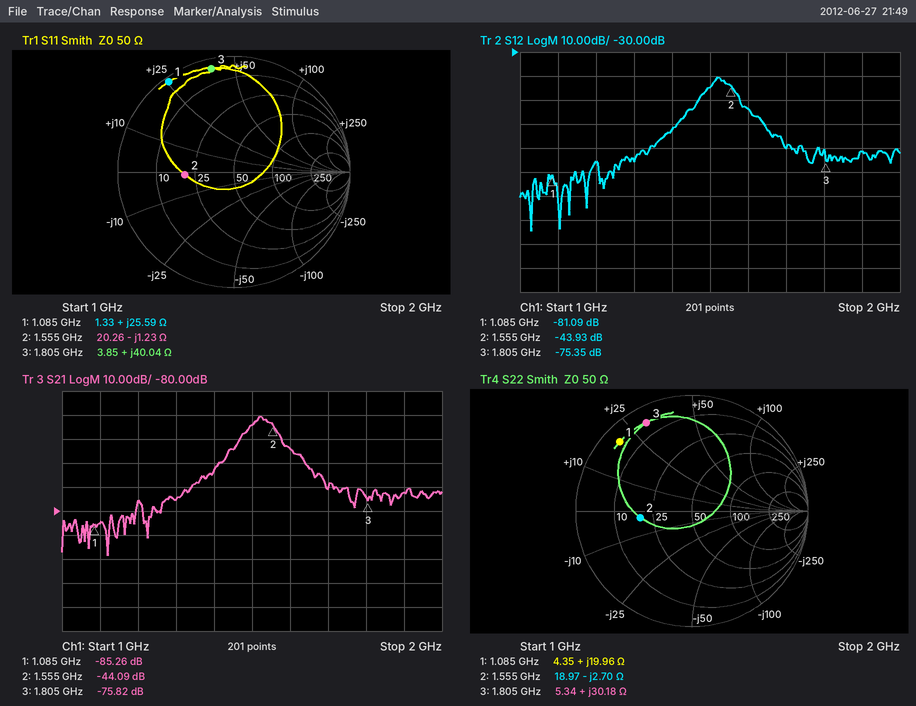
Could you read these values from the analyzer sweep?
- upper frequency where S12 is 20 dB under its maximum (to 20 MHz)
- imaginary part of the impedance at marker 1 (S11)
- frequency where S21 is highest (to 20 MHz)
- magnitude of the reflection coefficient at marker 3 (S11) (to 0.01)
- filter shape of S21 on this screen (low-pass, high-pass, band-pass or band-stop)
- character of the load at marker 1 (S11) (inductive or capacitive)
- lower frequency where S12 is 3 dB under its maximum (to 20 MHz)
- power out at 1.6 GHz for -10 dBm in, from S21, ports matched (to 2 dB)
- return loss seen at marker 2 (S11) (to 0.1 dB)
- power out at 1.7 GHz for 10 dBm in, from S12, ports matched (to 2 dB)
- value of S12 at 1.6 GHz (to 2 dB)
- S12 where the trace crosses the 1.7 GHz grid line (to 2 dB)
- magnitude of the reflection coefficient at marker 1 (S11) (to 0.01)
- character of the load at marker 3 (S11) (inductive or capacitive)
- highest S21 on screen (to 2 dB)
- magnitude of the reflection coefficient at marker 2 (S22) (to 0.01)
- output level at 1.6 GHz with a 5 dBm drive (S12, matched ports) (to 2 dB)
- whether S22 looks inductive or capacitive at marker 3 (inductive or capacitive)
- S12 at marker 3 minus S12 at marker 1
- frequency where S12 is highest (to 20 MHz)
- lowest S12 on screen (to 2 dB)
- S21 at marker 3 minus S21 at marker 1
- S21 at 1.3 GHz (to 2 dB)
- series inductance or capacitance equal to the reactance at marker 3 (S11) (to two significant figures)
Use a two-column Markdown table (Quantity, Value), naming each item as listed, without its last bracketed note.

| Quantity | Value |
|---|---|
| upper frequency where S12 is 20 dB under its maximum | 1.64 GHz |
| imaginary part of the impedance at marker 1 | +25.59 Ω |
| frequency where S21 is highest | 1.52 GHz |
| magnitude of the reflection coefficient at marker 3 (S11) | 0.91 |
| filter shape of S21 on this screen | band-pass |
| character of the load at marker 1 (S11) | inductive |
| lower frequency where S12 is 3 dB under its maximum | 1.50 GHz |
| power out at 1.6 GHz for -10 dBm in, from S21, ports matched | -64 dBm |
| return loss seen at marker 2 (S11) | 7.5 dB |
| power out at 1.7 GHz for 10 dBm in, from S12, ports matched | -60 dBm |
| value of S12 at 1.6 GHz | -54 dB |
| S12 where the trace crosses the 1.7 GHz grid line | -70 dB |
| magnitude of the reflection coefficient at marker 1 (S11) | 0.96 |
| character of the load at marker 3 (S11) | inductive |
| highest S21 on screen | -40 dB |
| magnitude of the reflection coefficient at marker 2 (S22) | 0.45 |
| output level at 1.6 GHz with a 5 dBm drive (S12, matched ports) | -48 dBm |
| whether S22 looks inductive or capacitive at marker 3 | inductive |
| S12 at marker 3 minus S12 at marker 1 | 5.74 dB |
| frequency where S12 is highest | 1.52 GHz |
| lowest S12 on screen | -104 dB |
| S21 at marker 3 minus S21 at marker 1 | 9.44 dB |
| S21 at 1.3 GHz | -76 dB |
| series inductance or capacitance equal to the reactance at marker 3 (S11) | 3.5 nH |
